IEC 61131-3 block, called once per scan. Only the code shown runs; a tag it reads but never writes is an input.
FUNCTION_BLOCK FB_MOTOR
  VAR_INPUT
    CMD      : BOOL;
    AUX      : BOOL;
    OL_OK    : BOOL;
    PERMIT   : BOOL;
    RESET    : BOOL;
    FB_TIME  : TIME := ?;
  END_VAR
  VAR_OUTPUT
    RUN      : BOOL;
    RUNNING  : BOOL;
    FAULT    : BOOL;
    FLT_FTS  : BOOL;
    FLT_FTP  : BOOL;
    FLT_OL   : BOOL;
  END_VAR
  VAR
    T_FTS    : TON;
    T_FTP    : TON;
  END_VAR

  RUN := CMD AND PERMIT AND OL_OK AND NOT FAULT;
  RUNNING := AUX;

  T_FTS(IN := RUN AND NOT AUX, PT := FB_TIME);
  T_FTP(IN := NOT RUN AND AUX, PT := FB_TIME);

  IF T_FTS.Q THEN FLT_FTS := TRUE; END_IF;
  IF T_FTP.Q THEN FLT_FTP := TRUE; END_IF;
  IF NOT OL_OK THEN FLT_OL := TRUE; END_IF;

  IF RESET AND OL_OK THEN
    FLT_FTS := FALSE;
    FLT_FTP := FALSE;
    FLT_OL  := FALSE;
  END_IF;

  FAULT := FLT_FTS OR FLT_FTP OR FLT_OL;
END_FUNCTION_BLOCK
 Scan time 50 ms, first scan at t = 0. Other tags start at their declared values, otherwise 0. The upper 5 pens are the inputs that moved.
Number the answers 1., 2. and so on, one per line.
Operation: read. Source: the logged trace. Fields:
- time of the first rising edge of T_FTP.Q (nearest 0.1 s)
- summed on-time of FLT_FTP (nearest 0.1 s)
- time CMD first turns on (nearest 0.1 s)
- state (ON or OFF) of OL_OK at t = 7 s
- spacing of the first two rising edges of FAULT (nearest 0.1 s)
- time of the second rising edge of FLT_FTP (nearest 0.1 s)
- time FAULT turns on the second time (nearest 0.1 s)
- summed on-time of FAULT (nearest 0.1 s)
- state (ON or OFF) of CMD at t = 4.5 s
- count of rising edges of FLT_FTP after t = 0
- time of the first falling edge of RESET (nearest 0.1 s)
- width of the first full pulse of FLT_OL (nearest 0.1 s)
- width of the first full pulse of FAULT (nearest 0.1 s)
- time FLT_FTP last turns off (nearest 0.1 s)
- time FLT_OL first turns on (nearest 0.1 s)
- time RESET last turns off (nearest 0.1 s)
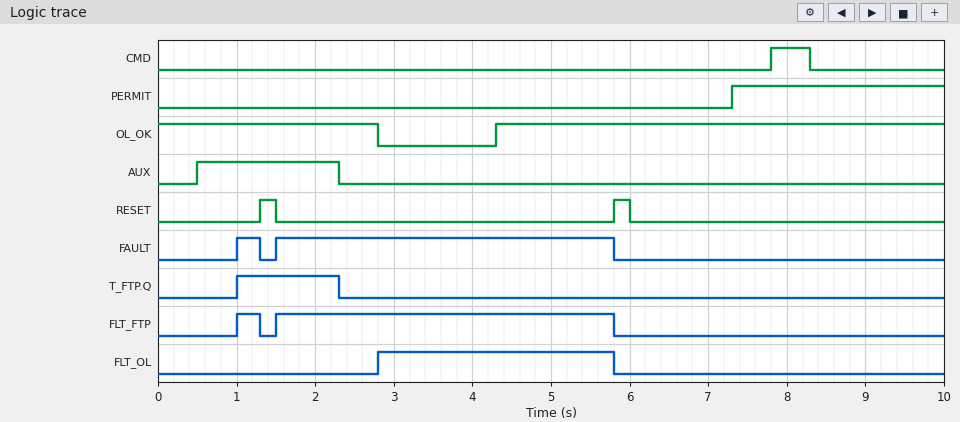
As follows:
1. 1.0 s
2. 4.6 s
3. 7.8 s
4. ON
5. 0.5 s
6. 1.5 s
7. 1.5 s
8. 4.6 s
9. OFF
10. 2
11. 1.5 s
12. 3.0 s
13. 0.3 s
14. 5.8 s
15. 2.8 s
16. 6.0 s
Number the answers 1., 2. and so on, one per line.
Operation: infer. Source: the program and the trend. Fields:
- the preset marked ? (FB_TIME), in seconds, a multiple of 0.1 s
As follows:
1. 0.5 s
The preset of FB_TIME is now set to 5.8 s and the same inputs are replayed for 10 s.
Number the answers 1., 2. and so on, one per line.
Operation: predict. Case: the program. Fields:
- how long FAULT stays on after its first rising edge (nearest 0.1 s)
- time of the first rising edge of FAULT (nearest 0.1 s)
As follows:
1. 3.0 s
2. 2.8 s
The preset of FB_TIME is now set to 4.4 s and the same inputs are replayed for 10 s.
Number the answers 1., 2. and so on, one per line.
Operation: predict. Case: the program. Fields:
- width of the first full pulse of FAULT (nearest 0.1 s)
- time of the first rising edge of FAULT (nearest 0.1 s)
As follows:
1. 3.0 s
2. 2.8 s
